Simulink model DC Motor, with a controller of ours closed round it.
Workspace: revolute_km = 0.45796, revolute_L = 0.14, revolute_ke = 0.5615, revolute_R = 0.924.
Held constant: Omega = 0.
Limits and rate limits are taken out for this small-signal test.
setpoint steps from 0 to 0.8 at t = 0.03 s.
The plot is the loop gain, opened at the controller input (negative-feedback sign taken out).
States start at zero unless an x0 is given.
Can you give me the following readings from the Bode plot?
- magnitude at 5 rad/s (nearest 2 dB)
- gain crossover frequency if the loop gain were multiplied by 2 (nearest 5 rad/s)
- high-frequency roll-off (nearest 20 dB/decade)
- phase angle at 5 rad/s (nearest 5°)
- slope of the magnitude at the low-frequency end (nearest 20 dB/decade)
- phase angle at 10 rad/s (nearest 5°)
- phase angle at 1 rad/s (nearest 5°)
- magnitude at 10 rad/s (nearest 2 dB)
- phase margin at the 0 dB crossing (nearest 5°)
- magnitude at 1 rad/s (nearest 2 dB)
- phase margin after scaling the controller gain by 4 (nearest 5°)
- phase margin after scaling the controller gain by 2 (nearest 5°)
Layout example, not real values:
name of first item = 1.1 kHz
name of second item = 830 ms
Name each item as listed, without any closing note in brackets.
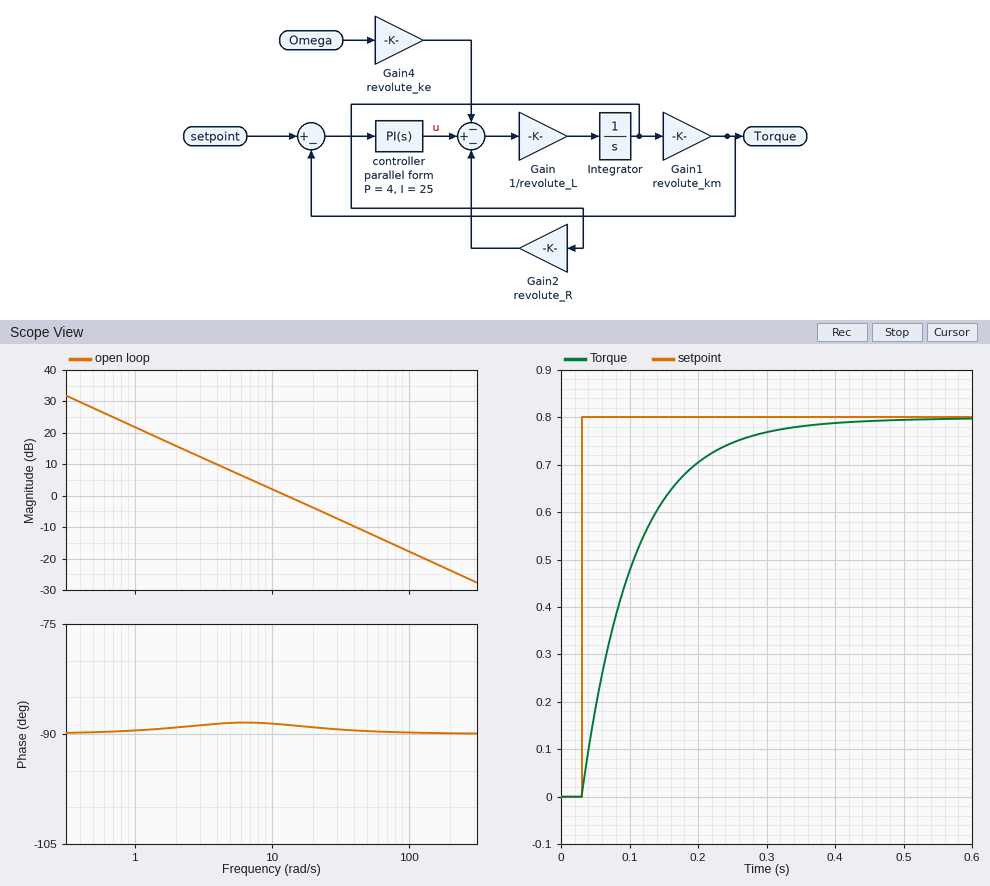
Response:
magnitude at 5 rad/s = 8 dB
gain crossover frequency if the loop gain were multiplied by 2 = 25 rad/s
high-frequency roll-off = -20 dB/decade
phase angle at 5 rad/s = -90°
slope of the magnitude at the low-frequency end = -20 dB/decade
phase angle at 10 rad/s = -90°
phase angle at 1 rad/s = -90°
magnitude at 10 rad/s = 2 dB
phase margin at the 0 dB crossing = 90°
magnitude at 1 rad/s = 22 dB
phase margin after scaling the controller gain by 4 = 90°
phase margin after scaling the controller gain by 2 = 90°
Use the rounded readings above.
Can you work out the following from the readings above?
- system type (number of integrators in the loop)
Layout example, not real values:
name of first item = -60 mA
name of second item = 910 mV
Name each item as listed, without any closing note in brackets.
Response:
system type = 1
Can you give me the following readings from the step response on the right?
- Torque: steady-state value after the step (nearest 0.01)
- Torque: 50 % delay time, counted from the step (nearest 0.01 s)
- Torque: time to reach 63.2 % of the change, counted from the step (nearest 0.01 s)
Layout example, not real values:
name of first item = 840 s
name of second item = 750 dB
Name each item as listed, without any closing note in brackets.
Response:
Torque: steady-state value after the step = 0.80
Torque: 50 % delay time, counted from the step = 0.05 s
Torque: time to reach 63.2 % of the change, counted from the step = 0.08 s
